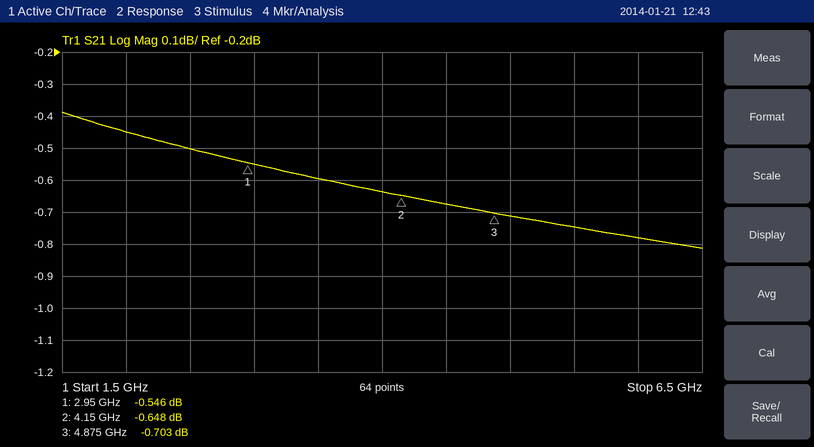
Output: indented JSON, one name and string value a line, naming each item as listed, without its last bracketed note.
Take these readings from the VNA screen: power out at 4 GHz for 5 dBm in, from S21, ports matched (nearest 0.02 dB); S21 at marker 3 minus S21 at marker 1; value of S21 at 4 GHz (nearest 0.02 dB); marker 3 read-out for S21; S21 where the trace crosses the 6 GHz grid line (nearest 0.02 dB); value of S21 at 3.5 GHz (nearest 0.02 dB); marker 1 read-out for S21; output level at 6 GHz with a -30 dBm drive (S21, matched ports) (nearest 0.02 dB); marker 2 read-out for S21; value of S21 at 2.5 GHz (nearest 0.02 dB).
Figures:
{
  "power out at 4 GHz for 5 dBm in, from S21, ports matched": "4.36 dBm",
  "S21 at marker 3 minus S21 at marker 1": "-0.157 dB",
  "value of S21 at 4 GHz": "-0.64 dB",
  "marker 3 read-out for S21": "-0.703 dB",
  "S21 where the trace crosses the 6 GHz grid line": "-0.78 dB",
  "value of S21 at 3.5 GHz": "-0.60 dB",
  "marker 1 read-out for S21": "-0.546 dB",
  "output level at 6 GHz with a -30 dBm drive (S21, matched ports)": "-30.78 dBm",
  "marker 2 read-out for S21": "-0.648 dB",
  "value of S21 at 2.5 GHz": "-0.50 dB"
}
